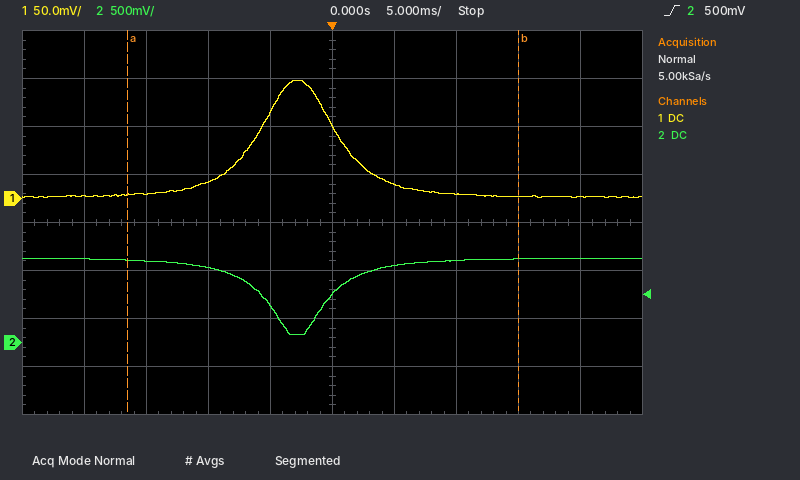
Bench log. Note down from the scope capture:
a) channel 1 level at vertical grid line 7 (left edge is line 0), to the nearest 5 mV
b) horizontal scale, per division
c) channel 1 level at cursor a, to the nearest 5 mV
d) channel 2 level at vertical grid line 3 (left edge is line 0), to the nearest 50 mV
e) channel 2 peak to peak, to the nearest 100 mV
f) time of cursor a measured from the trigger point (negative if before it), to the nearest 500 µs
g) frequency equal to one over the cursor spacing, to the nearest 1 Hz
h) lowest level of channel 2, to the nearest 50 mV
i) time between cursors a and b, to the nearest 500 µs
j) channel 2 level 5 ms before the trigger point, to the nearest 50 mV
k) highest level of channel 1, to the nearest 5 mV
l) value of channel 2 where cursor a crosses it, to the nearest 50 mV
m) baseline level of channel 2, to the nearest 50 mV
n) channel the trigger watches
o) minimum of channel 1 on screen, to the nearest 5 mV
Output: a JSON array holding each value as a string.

["5 mV", "5 ms", "5 mV", "800 mV", "800 mV", "-16.5 ms", "32 Hz", "100 mV", "31.5 ms", "400 mV", "125 mV", "850 mV", "850 mV", "channel 2", "0 mV"]
